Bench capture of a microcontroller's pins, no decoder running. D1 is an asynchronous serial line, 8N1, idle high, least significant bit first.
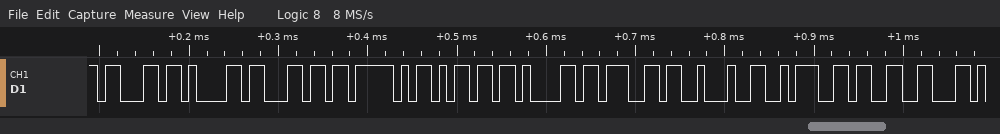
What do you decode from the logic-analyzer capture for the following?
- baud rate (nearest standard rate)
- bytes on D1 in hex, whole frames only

115200 baud
0x63 0x61 0x6C 0x5F 0x6D 0x61 0x67 0x22 0x3A 0x33
